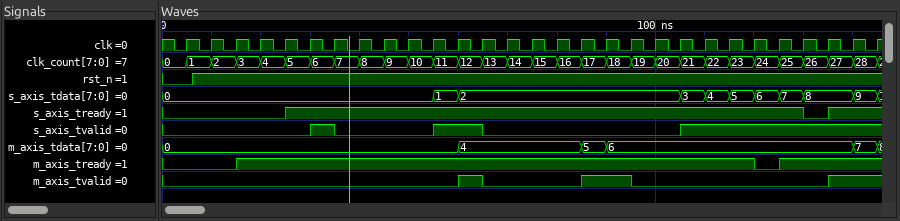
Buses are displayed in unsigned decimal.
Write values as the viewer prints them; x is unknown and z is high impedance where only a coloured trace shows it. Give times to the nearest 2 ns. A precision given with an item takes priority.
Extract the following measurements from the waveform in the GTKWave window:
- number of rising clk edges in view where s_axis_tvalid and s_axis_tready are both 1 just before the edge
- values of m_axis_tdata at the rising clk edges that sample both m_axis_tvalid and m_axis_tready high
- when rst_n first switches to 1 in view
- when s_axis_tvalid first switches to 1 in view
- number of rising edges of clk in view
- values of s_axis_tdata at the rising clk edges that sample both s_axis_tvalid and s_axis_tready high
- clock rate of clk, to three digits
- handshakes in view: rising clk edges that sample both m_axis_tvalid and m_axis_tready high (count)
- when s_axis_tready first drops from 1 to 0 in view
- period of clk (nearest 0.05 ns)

10
4, 5, 6, 6, 7
6 ns
30 ns
29
0, 1, 2, 3, 4, 5, 6, 7, 8, 9
200 MHz
5
130 ns
5 ns
